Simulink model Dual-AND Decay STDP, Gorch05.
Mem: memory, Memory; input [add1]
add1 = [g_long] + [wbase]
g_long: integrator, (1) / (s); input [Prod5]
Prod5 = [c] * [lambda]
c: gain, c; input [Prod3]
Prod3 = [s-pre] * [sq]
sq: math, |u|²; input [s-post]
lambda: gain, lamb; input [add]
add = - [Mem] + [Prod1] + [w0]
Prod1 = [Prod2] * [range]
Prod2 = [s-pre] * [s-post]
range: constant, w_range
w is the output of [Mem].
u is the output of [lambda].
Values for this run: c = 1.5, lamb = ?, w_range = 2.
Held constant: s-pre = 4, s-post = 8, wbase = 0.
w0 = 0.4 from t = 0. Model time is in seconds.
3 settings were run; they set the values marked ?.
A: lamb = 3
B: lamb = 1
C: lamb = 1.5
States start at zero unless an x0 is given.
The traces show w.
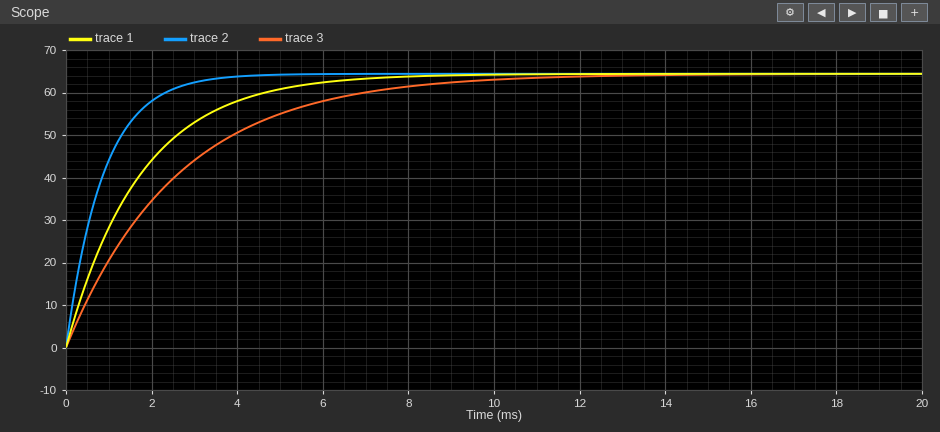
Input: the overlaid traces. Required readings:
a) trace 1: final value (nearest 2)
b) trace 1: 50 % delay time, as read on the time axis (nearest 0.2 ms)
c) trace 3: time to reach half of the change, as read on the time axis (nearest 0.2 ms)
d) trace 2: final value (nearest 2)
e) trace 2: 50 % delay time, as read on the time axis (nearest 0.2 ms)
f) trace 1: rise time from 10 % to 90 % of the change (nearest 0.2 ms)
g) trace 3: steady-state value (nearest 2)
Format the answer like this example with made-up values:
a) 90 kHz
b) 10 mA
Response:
a) 64
b) 1.2 ms
c) 1.8 ms
d) 64
e) 0.6 ms
f) 3.8 ms
g) 64
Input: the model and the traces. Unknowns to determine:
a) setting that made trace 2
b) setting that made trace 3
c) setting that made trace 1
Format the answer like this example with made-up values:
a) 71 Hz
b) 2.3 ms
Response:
a) A
b) B
c) C
